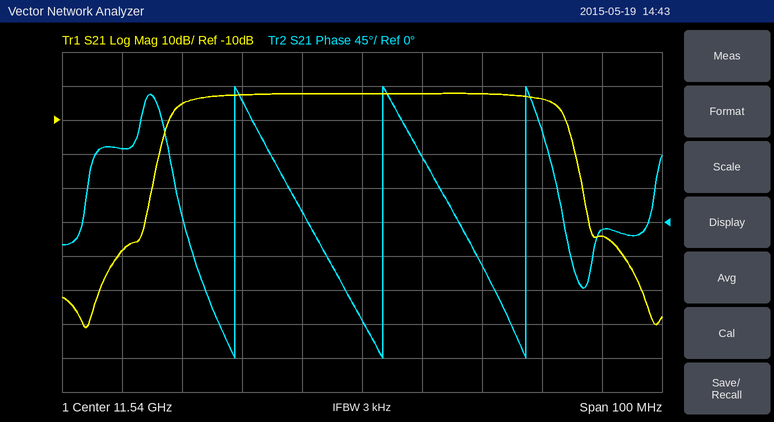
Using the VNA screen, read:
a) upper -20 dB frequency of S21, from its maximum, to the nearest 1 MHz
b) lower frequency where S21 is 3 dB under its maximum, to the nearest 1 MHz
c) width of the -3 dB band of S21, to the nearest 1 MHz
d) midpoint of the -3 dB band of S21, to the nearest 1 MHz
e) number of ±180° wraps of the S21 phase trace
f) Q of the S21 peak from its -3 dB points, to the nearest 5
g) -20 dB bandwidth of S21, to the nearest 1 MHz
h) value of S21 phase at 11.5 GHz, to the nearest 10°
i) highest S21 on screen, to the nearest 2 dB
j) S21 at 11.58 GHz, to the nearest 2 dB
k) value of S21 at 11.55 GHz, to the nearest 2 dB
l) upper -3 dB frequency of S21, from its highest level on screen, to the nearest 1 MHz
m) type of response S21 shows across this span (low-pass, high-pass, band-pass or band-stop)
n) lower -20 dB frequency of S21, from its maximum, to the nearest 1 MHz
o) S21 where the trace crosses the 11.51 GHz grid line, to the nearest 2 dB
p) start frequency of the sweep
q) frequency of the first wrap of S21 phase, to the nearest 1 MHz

11.576 GHz
11.510 GHz
62 MHz
11.541 GHz
3
185
70 MHz
100°
-2 dB
-44 dB
-2 dB
11.572 GHz
band-pass
11.506 GHz
-6 dB
11.49 GHz
11.519 GHz
